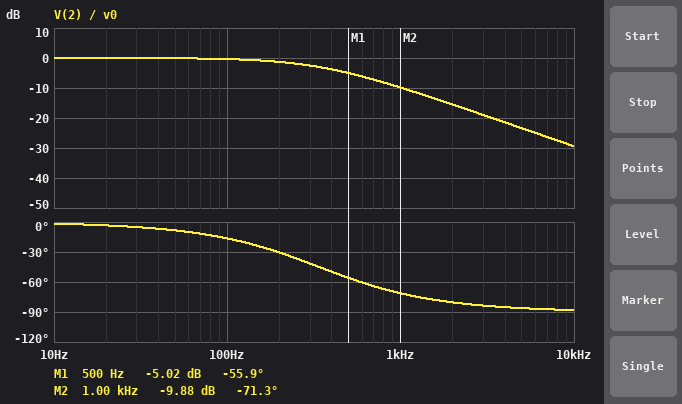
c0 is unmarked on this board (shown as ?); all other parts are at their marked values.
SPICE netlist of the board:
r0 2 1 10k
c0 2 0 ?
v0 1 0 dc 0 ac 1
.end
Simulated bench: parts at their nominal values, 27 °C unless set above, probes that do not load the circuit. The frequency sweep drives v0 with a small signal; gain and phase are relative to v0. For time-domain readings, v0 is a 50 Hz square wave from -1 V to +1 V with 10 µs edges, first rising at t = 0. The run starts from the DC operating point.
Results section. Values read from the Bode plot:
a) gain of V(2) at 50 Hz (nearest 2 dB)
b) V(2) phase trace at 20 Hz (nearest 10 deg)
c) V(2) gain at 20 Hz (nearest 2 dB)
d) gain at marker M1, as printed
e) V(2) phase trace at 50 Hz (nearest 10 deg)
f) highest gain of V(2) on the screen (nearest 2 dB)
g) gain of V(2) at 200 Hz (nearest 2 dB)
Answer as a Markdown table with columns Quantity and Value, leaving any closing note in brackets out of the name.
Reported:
| Quantity | Value |
|---|---|
| gain of V(2) at 50 Hz | 0 dB |
| V(2) phase trace at 20 Hz | 0 deg |
| V(2) gain at 20 Hz | 0 dB |
| gain at marker M1, as printed | -5.02 dB |
| V(2) phase trace at 50 Hz | -10 deg |
| highest gain of V(2) on the screen | 0 dB |
| gain of V(2) at 200 Hz | -2 dB |
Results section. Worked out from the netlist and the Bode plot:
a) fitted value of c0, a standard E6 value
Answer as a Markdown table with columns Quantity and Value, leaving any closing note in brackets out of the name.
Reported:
| Quantity | Value |
|---|---|
| fitted value of c0, a standard E6 value | 47 nF |
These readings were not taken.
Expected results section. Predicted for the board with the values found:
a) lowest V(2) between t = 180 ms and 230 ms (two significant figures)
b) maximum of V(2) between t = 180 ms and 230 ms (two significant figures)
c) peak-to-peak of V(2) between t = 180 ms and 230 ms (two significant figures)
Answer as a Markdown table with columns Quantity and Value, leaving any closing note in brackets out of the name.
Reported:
| Quantity | Value |
|---|---|
| lowest V(2) between t = 180 ms and 230 ms | -1.0 V |
| maximum of V(2) between t = 180 ms and 230 ms | 1.0 V |
| peak-to-peak of V(2) between t = 180 ms and 230 ms | 2.0 V |
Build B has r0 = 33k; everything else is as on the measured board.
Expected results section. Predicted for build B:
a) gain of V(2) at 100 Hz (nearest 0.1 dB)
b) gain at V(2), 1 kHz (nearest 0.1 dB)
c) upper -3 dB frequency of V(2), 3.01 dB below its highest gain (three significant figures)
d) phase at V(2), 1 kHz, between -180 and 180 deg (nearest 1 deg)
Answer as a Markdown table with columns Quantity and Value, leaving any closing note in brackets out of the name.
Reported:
| Quantity | Value |
|---|---|
| gain of V(2) at 100 Hz | -2.9 dB |
| gain at V(2), 1 kHz | -19.8 dB |
| upper -3 dB frequency of V(2), 3.01 dB below its highest gain | 103 Hz |
| phase at V(2), 1 kHz, between -180 and 180 deg | -84 deg |
